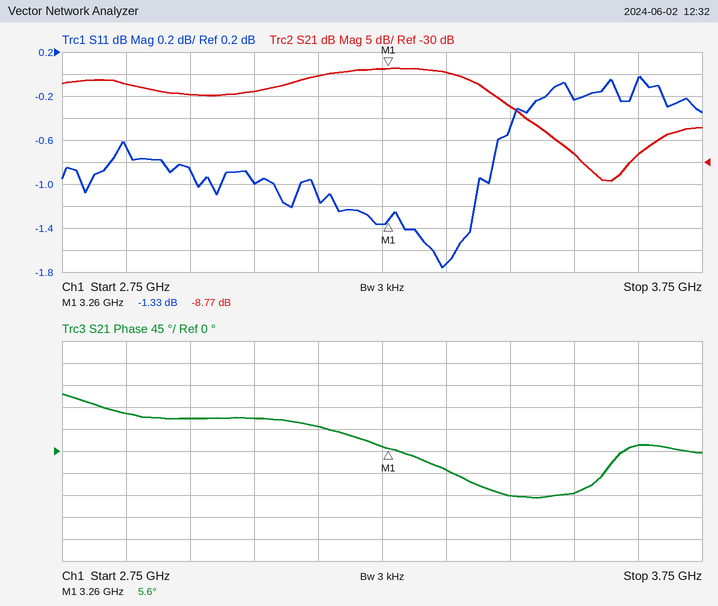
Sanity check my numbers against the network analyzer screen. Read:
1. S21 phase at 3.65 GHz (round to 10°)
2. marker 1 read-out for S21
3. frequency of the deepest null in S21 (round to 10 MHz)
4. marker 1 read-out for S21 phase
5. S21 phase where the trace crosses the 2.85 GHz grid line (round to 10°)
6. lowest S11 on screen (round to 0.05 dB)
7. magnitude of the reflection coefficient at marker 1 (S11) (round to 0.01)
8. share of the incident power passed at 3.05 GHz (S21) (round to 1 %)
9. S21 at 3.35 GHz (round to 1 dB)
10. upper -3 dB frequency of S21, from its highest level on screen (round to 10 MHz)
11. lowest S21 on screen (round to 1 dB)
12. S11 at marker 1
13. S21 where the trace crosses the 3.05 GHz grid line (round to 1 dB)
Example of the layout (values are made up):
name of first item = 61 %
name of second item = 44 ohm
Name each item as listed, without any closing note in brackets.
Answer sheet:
S21 phase at 3.65 GHz = 10°
marker 1 read-out for S21 = -8.77 dB
frequency of the deepest null in S21 = 3.61 GHz
marker 1 read-out for S21 phase = 5.6°
S21 phase where the trace crosses the 2.85 GHz grid line = 80°
lowest S11 on screen = -1.75 dB
magnitude of the reflection coefficient at marker 1 (S11) = 0.86
share of the incident power passed at 3.05 GHz (S21) = 4 %
S21 at 3.35 GHz = -10 dB
upper -3 dB frequency of S21, from its highest level on screen = 3.39 GHz
lowest S21 on screen = -34 dB
S11 at marker 1 = -1.33 dB
S21 where the trace crosses the 3.05 GHz grid line = -14 dB
